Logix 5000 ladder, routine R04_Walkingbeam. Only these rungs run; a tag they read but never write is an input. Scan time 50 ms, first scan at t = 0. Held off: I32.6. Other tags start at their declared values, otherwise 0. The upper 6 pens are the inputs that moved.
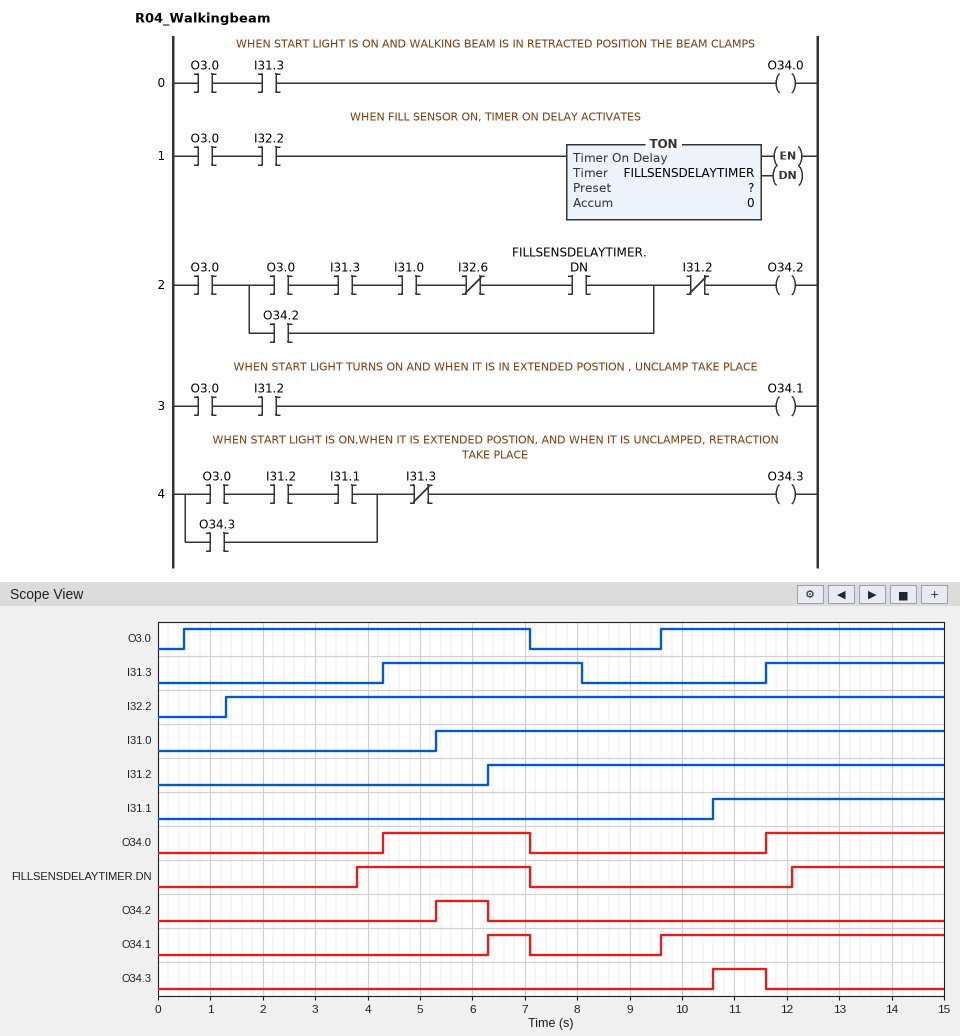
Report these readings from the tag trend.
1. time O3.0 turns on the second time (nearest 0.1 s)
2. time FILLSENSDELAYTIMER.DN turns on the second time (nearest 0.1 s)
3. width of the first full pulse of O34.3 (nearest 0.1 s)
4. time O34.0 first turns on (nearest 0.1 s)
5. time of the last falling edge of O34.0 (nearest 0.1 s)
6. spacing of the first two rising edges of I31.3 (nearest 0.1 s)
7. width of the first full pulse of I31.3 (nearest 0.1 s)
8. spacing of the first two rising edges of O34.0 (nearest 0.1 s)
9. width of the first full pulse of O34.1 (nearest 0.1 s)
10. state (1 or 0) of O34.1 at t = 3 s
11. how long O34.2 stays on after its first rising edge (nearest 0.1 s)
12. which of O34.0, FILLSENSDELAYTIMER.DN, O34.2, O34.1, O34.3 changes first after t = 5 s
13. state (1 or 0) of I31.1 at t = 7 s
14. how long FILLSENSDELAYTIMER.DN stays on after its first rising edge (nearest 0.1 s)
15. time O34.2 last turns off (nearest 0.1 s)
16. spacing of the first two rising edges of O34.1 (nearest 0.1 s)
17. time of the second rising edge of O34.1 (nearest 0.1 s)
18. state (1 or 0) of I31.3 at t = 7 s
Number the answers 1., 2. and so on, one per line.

1. 9.6 s
2. 12.1 s
3. 1.0 s
4. 4.3 s
5. 7.1 s
6. 7.3 s
7. 3.8 s
8. 7.3 s
9. 0.8 s
10. 0
11. 1.0 s
12. O34.2
13. 0
14. 3.3 s
15. 6.3 s
16. 3.3 s
17. 9.6 s
18. 1
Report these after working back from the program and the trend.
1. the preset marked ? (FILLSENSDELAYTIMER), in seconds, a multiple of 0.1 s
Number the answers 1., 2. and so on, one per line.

1. 2.5 s
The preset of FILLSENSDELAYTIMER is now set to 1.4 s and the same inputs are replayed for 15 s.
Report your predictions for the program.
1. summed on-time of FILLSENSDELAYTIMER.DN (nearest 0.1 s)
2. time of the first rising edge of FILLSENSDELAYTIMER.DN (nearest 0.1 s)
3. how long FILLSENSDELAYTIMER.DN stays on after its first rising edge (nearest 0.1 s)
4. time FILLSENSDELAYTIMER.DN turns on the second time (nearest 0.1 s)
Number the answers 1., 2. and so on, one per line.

1. 8.4 s
2. 2.7 s
3. 4.4 s
4. 11.0 s
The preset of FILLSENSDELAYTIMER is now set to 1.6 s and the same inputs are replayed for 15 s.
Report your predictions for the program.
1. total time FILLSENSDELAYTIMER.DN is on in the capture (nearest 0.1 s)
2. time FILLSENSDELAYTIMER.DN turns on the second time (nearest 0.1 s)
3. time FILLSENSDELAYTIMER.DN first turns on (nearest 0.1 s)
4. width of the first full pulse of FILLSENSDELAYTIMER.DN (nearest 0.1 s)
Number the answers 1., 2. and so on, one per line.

1. 8.0 s
2. 11.2 s
3. 2.9 s
4. 4.2 s
